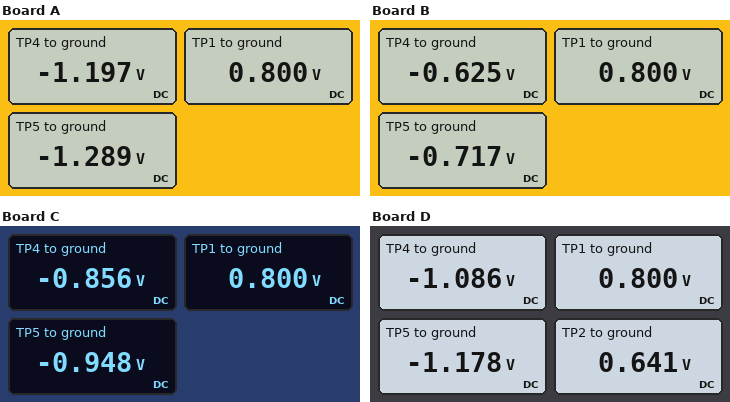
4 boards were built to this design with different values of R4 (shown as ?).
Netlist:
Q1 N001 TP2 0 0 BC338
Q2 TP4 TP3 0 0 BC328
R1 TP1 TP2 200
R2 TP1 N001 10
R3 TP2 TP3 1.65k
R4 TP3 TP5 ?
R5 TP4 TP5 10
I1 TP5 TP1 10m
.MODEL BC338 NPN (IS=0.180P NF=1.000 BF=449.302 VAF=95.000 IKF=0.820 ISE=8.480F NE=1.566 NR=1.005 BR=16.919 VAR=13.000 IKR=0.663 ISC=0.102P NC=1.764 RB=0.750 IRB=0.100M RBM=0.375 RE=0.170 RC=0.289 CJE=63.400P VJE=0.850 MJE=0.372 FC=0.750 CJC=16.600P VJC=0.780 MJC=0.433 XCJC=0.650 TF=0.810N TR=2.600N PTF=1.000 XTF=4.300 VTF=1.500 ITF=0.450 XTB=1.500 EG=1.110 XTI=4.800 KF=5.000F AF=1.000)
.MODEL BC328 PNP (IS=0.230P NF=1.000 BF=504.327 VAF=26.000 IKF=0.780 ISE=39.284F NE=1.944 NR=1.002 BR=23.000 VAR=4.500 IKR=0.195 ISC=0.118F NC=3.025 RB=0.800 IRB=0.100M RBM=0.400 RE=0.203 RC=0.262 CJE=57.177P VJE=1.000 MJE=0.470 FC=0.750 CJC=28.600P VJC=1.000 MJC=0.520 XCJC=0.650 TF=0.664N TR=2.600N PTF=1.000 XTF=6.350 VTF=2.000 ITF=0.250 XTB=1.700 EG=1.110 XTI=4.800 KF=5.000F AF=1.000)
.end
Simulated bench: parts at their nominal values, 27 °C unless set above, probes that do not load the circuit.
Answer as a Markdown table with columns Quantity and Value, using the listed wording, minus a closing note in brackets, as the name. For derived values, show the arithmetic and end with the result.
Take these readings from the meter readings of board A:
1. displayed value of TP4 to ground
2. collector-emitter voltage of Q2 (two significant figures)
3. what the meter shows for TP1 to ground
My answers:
| Quantity | Value |
|---|---|
| displayed value of TP4 to ground | -1.197 V |
| collector-emitter voltage of Q2 | -1.197 V = -1.2 V |
| what the meter shows for TP1 to ground | 0.800 V |
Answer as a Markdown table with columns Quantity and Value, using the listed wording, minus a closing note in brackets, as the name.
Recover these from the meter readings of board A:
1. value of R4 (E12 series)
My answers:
| Quantity | Value |
|---|---|
| value of R4 | 820 Ω |
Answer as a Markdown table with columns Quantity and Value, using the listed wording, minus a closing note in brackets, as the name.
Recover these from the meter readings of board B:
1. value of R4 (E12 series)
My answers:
| Quantity | Value |
|---|---|
| value of R4 | 100 Ω |
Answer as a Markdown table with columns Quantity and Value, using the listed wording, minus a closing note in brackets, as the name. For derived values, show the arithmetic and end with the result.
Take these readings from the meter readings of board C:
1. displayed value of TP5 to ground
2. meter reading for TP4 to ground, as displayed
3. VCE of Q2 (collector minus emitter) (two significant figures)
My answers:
| Quantity | Value |
|---|---|
| displayed value of TP5 to ground | -0.948 V |
| meter reading for TP4 to ground, as displayed | -0.856 V |
| VCE of Q2 (collector minus emitter) | -856 mV = -860 mV |
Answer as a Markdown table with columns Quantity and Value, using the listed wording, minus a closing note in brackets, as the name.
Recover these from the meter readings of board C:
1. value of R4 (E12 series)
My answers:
| Quantity | Value |
|---|---|
| value of R4 | 390 Ω |
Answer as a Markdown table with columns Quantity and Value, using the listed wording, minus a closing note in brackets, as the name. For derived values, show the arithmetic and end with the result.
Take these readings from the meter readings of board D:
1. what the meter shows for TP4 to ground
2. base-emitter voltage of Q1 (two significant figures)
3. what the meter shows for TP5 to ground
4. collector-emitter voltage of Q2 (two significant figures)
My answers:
| Quantity | Value |
|---|---|
| what the meter shows for TP4 to ground | -1.086 V |
| base-emitter voltage of Q1 | 641 mV = 640 mV |
| what the meter shows for TP5 to ground | -1.178 V |
| collector-emitter voltage of Q2 | -1.086 V = -1.1 V |
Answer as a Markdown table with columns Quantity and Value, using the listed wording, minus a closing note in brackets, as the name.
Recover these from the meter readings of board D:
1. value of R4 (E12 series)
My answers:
| Quantity | Value |
|---|---|
| value of R4 | 680 Ω |
